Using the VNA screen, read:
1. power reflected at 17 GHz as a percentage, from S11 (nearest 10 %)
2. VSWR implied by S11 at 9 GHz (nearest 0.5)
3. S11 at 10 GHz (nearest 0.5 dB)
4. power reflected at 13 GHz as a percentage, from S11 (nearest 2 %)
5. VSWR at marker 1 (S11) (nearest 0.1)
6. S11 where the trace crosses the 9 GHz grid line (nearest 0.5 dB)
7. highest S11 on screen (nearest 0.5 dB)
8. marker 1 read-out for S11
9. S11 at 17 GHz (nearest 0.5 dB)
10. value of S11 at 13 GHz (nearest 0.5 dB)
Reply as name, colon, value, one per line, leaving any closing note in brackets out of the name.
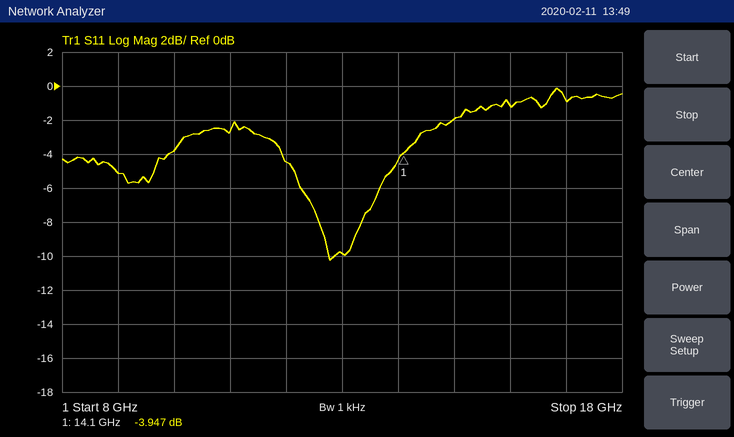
power reflected at 17 GHz as a percentage, from S11: 80 %
VSWR implied by S11 at 9 GHz: 3.5
S11 at 10 GHz: -4.0 dB
power reflected at 13 GHz as a percentage, from S11: 10 %
VSWR at marker 1 (S11): 4.5
S11 where the trace crosses the 9 GHz grid line: -5.0 dB
highest S11 on screen: 0.0 dB
marker 1 read-out for S11: -3.947 dB
S11 at 17 GHz: -1.0 dB
value of S11 at 13 GHz: -10.0 dB
